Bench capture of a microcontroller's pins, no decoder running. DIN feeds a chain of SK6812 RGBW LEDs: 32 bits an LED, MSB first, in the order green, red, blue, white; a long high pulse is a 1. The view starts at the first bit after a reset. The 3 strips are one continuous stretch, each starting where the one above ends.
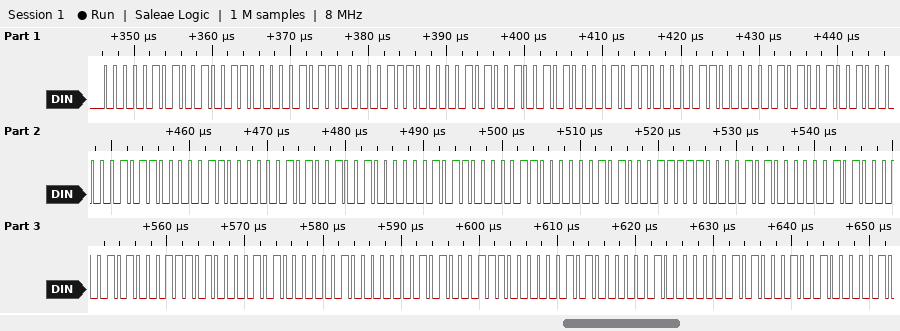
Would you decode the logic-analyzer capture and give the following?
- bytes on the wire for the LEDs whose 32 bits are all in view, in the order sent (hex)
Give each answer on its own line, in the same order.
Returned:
05 26 0B 07 05 25 0B 06 05 24 0B 06 05 24 0B 06 05 1F 0A 05 05 1D 0A 04 05 1C 0A 04
